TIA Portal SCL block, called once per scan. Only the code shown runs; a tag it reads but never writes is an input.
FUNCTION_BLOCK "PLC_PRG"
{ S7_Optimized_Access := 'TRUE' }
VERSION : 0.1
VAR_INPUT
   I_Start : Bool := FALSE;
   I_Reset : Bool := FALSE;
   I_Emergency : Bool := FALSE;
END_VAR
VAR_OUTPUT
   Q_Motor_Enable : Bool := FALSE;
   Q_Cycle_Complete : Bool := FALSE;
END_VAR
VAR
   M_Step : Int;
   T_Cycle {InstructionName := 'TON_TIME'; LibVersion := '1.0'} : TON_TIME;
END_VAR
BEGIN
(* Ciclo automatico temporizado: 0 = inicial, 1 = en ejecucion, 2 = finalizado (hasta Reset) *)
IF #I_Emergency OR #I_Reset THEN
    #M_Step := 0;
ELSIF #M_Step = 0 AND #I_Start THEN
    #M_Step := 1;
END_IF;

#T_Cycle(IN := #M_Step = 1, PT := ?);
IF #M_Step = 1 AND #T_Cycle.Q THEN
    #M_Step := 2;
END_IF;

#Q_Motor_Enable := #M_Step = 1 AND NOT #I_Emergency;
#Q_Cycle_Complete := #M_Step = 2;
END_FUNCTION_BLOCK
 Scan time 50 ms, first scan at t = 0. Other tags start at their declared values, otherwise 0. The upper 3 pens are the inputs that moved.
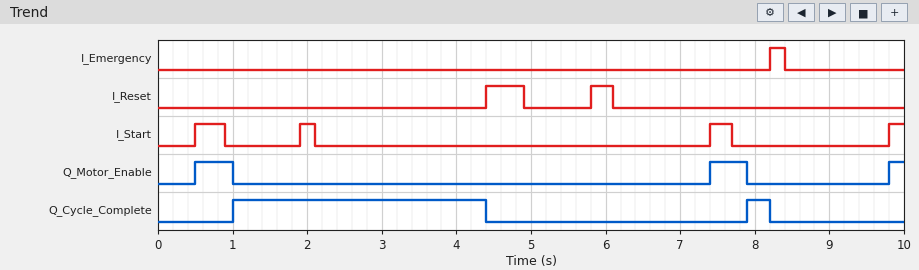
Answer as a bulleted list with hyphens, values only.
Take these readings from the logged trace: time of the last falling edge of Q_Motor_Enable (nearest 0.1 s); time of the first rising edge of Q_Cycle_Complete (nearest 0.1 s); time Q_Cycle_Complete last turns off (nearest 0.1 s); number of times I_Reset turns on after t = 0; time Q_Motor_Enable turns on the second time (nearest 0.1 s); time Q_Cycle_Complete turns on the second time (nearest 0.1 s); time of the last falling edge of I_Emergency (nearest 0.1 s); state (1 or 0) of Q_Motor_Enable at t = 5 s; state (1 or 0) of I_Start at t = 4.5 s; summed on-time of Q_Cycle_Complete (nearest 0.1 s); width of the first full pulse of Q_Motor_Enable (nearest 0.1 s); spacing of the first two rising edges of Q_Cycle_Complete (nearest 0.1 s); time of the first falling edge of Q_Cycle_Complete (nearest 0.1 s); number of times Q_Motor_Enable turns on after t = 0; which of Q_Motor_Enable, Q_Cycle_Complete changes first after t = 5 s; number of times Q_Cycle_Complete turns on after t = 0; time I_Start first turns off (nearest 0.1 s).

- 7.9 s
- 1.0 s
- 8.2 s
- 2
- 7.4 s
- 7.9 s
- 8.4 s
- 0
- 0
- 3.7 s
- 0.5 s
- 6.9 s
- 4.4 s
- 3
- Q_Motor_Enable
- 2
- 0.9 s
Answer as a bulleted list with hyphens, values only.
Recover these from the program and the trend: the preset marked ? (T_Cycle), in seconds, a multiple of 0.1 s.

- 0.5 s
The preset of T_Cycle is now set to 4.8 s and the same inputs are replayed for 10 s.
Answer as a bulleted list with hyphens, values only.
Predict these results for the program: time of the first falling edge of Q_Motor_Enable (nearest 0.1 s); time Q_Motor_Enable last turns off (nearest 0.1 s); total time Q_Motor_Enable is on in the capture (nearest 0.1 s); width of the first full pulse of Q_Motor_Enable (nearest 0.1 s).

- 4.4 s
- 8.2 s
- 4.9 s
- 3.9 s
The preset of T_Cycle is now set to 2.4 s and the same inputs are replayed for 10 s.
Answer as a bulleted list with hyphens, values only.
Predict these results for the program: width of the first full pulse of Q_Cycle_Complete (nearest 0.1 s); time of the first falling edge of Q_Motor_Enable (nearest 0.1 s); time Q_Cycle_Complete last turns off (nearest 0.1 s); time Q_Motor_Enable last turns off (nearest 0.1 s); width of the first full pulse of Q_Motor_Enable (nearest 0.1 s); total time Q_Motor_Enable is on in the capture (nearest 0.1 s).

- 1.5 s
- 2.9 s
- 4.4 s
- 8.2 s
- 2.4 s
- 3.4 s
